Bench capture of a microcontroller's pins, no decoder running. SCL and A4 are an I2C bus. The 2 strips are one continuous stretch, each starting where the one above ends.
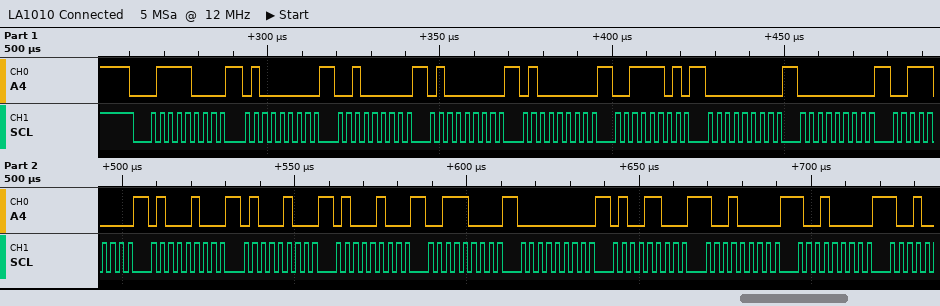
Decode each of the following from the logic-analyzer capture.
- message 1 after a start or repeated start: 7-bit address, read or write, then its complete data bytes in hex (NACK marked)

0x3C write: 40 20 40 40 3D 00 00 38 44 44 44 38 00 4C 90 90
